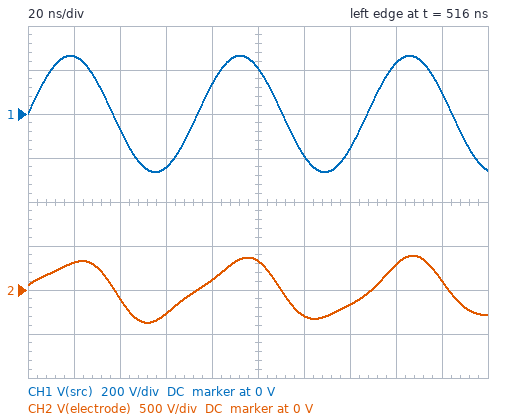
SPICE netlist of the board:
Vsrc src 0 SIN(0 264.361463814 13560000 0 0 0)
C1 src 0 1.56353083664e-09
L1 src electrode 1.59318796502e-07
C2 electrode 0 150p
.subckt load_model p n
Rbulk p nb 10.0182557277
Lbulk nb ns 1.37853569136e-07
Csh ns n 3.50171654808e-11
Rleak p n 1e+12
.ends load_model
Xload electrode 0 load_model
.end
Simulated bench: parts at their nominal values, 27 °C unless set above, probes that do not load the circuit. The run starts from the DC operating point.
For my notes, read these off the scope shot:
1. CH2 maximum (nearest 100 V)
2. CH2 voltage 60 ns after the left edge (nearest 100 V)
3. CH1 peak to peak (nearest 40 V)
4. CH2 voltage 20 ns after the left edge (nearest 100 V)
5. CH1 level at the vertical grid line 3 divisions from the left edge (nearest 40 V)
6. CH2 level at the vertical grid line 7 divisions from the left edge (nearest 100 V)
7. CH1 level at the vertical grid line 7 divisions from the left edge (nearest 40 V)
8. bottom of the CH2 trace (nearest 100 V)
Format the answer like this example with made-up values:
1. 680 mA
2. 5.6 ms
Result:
1. 400 V
2. -300 V
3. 520 V
4. 300 V
5. -240 V
6. -200 V
7. -160 V
8. -400 V
